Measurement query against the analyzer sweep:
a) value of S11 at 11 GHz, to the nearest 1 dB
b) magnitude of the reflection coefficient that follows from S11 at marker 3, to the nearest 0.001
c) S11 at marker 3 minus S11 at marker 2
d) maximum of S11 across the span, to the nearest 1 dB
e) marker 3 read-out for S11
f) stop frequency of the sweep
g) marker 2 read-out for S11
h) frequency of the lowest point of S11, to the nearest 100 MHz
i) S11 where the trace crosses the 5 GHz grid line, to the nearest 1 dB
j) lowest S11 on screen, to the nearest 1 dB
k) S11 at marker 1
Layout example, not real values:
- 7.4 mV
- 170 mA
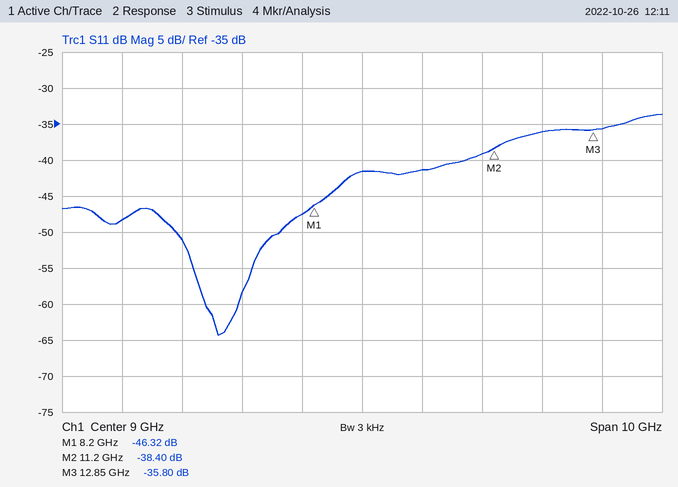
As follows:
- -39 dB
- 0.016
- 2.60 dB
- -34 dB
- -35.80 dB
- 14 GHz
- -38.40 dB
- 6.6 GHz
- -48 dB
- -64 dB
- -46.32 dB
